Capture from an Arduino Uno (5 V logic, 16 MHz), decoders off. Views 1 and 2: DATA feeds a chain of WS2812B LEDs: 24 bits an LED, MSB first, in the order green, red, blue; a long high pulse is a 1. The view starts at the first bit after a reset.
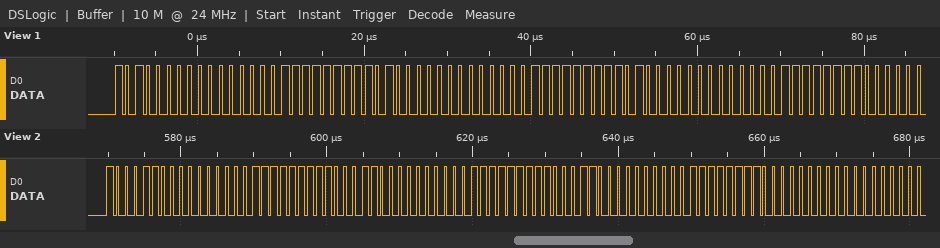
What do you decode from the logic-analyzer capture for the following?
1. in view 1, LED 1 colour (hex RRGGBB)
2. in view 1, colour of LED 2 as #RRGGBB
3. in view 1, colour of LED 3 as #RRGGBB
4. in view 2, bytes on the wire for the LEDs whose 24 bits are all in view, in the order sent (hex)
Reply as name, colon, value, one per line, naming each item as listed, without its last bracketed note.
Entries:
in view 1, LED 1 colour: #00A0FF
in view 1, colour of LED 2 as #RRGGBB: #00A0FF
in view 1, colour of LED 3 as #RRGGBB: #00A0FF
in view 2, bytes on the wire for the LEDs whose 24 bits are all in view, in the order sent: 8C 00 FF 8C 00 FF 8C 00 FF
